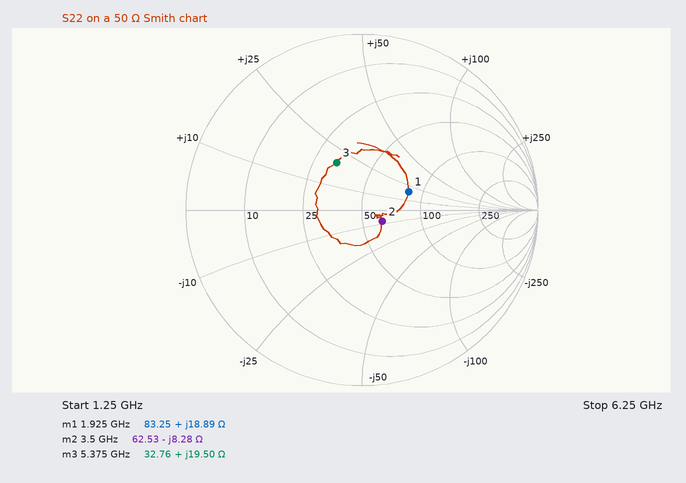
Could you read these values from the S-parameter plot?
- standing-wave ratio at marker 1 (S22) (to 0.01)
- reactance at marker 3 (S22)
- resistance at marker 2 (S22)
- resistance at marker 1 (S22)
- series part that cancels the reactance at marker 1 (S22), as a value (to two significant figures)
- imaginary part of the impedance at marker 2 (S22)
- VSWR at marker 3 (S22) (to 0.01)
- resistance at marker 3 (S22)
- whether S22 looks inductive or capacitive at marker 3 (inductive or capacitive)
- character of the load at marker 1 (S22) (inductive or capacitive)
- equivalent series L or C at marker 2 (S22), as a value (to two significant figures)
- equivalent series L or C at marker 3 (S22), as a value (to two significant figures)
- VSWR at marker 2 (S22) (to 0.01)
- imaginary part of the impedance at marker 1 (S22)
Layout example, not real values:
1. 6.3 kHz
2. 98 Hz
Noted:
1. 1.79
2. +19.50 Ω
3. 62.53 Ω
4. 83.25 Ω
5. 4.4 pF
6. -8.28 Ω
7. 1.88
8. 32.76 Ω
9. inductive
10. inductive
11. 5.5 pF
12. 580 pH
13. 1.31
14. +18.89 Ω
